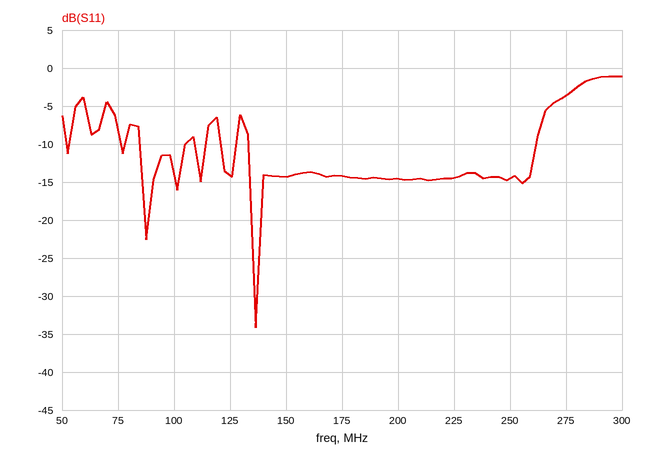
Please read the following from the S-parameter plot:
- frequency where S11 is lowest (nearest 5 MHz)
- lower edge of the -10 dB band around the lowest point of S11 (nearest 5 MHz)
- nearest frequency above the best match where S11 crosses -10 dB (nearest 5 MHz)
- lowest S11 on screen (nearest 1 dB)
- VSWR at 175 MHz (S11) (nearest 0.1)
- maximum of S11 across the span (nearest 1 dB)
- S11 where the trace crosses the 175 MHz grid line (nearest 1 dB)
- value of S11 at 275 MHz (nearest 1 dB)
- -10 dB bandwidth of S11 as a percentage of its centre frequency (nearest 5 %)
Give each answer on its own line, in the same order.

135 MHz
135 MHz
260 MHz
-34 dB
1.5
-1 dB
-14 dB
-4 dB
65 %
